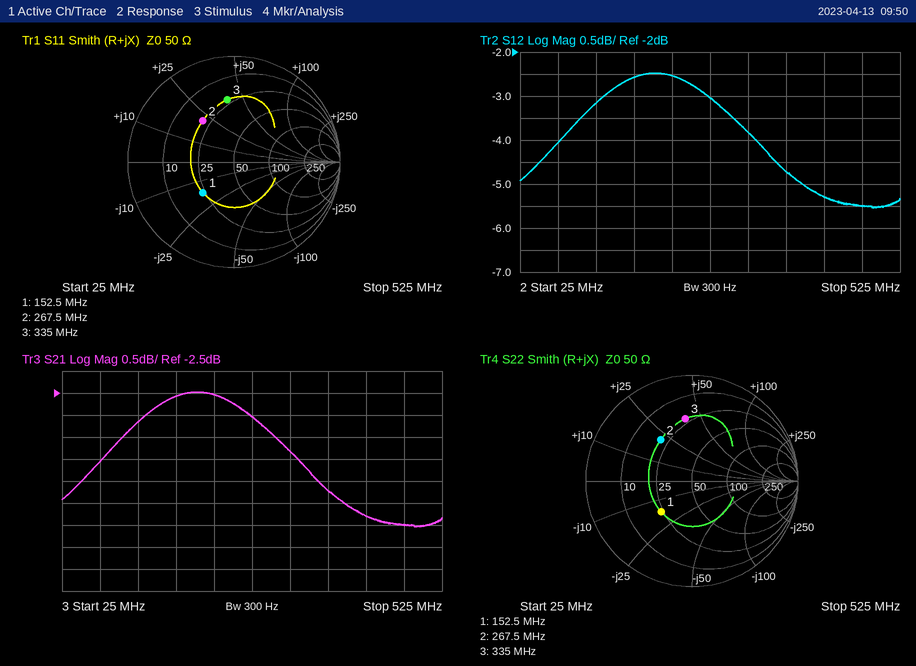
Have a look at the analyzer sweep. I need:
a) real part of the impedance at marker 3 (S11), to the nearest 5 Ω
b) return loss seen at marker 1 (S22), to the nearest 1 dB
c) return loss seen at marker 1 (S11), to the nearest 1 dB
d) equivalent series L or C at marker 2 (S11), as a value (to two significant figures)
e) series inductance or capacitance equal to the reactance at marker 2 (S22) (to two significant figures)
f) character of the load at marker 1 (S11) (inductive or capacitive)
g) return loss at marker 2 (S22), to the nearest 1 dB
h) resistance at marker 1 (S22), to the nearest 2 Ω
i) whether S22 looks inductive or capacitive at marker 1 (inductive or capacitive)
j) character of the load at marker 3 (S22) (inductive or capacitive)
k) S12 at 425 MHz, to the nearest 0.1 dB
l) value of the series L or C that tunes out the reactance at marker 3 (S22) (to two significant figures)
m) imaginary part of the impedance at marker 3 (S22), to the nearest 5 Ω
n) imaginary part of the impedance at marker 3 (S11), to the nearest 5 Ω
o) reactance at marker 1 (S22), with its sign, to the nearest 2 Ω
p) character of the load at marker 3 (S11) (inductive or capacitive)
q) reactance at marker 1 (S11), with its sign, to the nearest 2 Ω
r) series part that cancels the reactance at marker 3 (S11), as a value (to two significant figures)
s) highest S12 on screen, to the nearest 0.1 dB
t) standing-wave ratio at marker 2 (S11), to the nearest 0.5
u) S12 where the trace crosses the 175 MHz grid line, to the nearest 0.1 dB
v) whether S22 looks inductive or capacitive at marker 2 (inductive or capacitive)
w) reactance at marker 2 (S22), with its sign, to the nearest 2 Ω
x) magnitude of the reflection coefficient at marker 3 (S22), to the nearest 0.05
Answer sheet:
20 Ω
8 dB
8 dB
13 nH
13 nH
capacitive
6 dB
24 Ω
capacitive
inductive
-5.3 dB
12 pF
+40 Ω
+40 Ω
-16 Ω
inductive
-16 Ω
12 pF
-2.5 dB
3.0
-2.6 dB
inductive
+22 Ω
0.60
